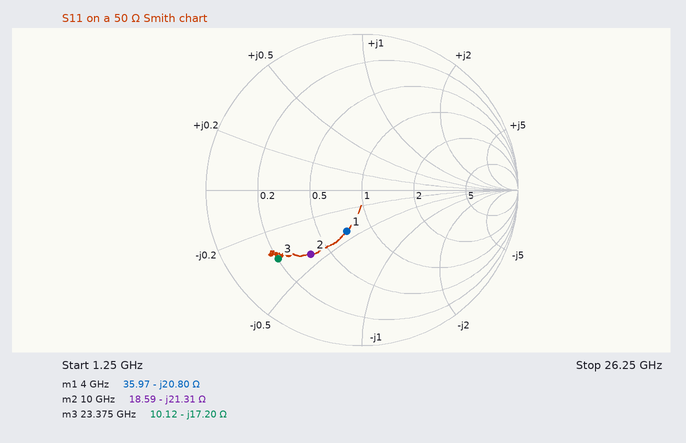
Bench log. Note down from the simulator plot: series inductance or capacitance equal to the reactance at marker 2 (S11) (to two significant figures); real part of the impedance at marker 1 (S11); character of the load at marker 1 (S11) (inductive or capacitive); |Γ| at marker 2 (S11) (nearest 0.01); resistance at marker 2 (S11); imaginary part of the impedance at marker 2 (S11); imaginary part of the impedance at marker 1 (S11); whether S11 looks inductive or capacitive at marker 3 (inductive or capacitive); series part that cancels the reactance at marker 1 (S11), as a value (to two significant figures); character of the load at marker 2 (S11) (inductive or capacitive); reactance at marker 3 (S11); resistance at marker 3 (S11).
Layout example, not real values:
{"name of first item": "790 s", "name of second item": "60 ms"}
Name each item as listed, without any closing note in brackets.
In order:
{"series inductance or capacitance equal to the reactance at marker 2 (S11)": "750 fF", "real part of the impedance at marker 1": "35.97 Ω", "character of the load at marker 1 (S11)": "capacitive", "|Γ| at marker 2 (S11)": "0.53", "resistance at marker 2": "18.59 Ω", "imaginary part of the impedance at marker 2": "-21.31 Ω", "imaginary part of the impedance at marker 1": "-20.80 Ω", "whether S11 looks inductive or capacitive at marker 3": "capacitive", "series part that cancels the reactance at marker 1 (S11), as a value": "830 pH", "character of the load at marker 2 (S11)": "capacitive", "reactance at marker 3": "-17.20 Ω", "resistance at marker 3": "10.12 Ω"}
